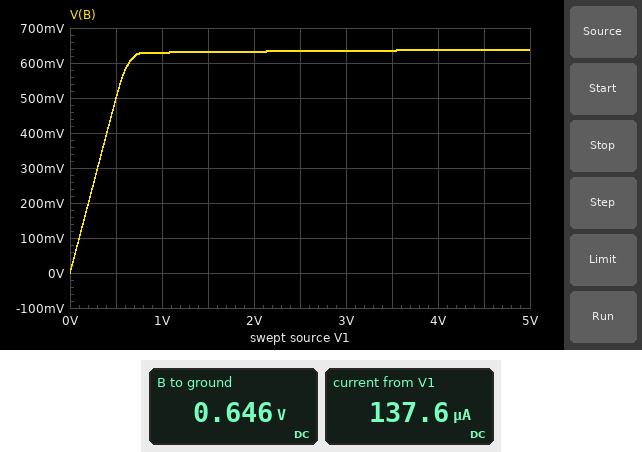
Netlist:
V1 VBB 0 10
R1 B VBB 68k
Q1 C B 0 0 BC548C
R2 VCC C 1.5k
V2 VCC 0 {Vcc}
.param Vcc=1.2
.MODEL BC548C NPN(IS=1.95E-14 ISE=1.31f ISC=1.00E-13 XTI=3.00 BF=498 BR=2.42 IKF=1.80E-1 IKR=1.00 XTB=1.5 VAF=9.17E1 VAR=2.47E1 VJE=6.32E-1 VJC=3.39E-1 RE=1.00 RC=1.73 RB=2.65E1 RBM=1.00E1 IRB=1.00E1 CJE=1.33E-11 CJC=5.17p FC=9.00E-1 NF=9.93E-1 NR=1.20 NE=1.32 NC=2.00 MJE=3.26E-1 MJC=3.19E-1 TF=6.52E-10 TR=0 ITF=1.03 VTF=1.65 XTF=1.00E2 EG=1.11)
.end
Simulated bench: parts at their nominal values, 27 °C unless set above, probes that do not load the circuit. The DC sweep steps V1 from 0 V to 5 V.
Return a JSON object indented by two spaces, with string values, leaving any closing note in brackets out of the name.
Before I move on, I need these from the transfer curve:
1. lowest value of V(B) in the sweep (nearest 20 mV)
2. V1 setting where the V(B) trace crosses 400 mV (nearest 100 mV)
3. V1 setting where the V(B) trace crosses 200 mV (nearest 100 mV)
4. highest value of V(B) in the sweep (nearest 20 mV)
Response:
{
  "lowest value of V(B) in the sweep": "0 V",
  "V1 setting where the V(B) trace crosses 400 mV": "400 mV",
  "V1 setting where the V(B) trace crosses 200 mV": "200 mV",
  "highest value of V(B) in the sweep": "640 mV"
}
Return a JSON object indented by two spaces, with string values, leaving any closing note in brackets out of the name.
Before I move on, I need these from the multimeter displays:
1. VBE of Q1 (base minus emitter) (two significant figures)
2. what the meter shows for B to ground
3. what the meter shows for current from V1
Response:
{
  "VBE of Q1 (base minus emitter)": "650 mV",
  "what the meter shows for B to ground": "0.646 V",
  "what the meter shows for current from V1": "137.6 µA"
}
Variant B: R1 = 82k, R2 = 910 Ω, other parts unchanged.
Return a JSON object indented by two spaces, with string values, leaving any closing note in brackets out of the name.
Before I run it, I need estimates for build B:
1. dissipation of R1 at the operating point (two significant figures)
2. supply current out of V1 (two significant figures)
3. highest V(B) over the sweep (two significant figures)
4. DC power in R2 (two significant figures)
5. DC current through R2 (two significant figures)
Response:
{
  "dissipation of R1 at the operating point": "1.1 mW",
  "supply current out of V1": "110 µA",
  "highest V(B) over the sweep": "650 mV",
  "DC power in R2": "1.8 mW",
  "DC current through R2": "1.4 mA"
}
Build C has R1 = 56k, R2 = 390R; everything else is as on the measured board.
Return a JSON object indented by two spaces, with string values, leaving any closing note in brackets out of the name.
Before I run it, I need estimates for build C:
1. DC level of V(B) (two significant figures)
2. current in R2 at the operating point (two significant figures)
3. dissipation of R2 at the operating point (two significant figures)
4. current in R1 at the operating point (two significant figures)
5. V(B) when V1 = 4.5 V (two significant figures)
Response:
{
  "DC level of V(B)": "680 mV",
  "current in R2 at the operating point": "3.2 mA",
  "dissipation of R2 at the operating point": "4.1 mW",
  "current in R1 at the operating point": "170 µA",
  "V(B) when V1 = 4.5 V": "670 mV"
}
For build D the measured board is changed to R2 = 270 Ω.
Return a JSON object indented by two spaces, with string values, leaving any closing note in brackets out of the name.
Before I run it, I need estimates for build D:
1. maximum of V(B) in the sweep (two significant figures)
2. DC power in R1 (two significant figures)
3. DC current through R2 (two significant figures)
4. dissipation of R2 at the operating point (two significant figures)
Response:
{
  "maximum of V(B) in the sweep": "680 mV",
  "DC power in R1": "1.3 mW",
  "DC current through R2": "4.6 mA",
  "dissipation of R2 at the operating point": "5.7 mW"
}
